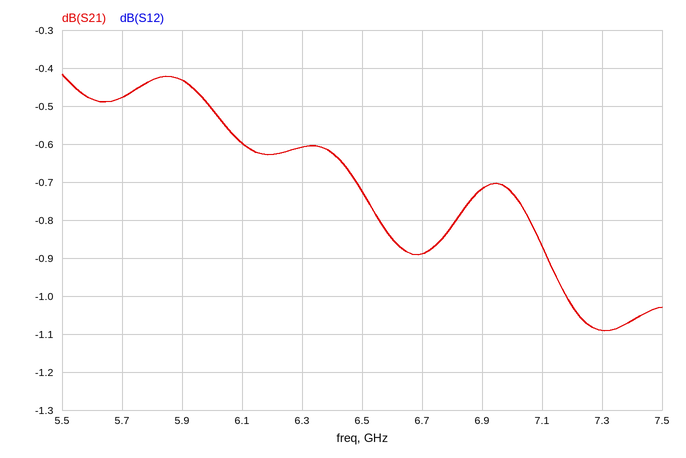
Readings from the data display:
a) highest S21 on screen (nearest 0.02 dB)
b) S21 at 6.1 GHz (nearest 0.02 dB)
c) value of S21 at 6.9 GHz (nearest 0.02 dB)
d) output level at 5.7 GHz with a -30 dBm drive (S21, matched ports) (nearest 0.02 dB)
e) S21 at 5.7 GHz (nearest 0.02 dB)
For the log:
-0.42 dB
-0.60 dB
-0.72 dB
-30.48 dBm
-0.48 dB
